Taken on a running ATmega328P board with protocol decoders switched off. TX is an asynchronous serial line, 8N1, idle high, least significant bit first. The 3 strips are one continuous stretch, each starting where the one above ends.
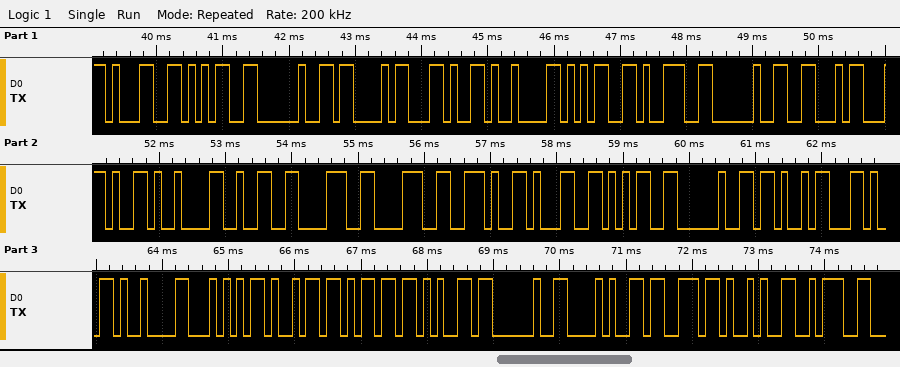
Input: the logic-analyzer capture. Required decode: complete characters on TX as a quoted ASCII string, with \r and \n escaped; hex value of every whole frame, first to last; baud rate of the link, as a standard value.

"15 C,\t59 F,\t288.15 K,\tTime (s):"
31 35 20 43 2C 09 35 39 20 46 2C 09 32 38 38 2E 31 35 20 4B 2C 09 54 69 6D 65 20 28 73 29 3A
9600 baud
